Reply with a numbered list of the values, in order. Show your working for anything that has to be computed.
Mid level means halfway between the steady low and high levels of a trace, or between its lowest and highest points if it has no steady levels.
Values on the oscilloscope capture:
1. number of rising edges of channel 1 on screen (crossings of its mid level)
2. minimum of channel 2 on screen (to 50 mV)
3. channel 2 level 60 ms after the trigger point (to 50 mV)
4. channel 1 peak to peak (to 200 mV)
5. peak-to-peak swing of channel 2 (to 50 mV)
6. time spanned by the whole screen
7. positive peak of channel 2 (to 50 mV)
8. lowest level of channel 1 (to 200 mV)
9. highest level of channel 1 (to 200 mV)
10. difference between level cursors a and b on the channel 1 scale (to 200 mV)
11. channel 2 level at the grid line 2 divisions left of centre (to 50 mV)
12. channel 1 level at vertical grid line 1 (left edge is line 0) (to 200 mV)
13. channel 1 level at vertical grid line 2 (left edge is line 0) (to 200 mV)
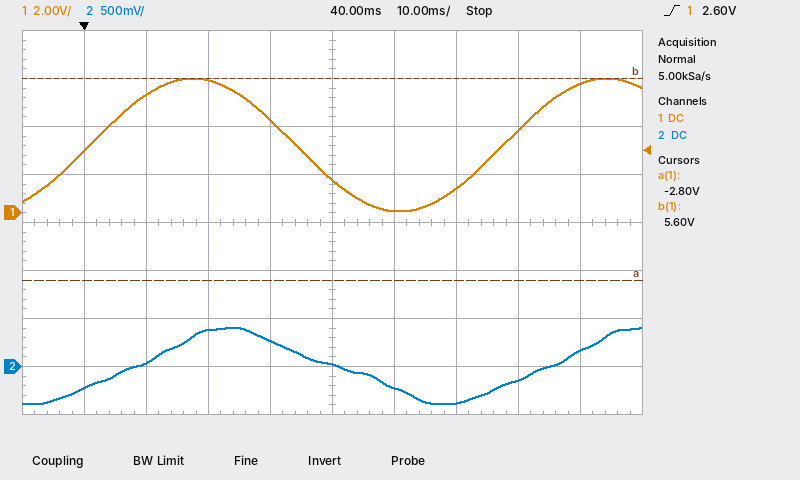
1. 2
2. -400 mV
3. -400 mV
4. 5.6 V − (0.0 V) = 5.6 V
5. 400 mV − (-400 mV) = 800 mV
6. 100 ms
7. 400 mV
8. 0.0 V
9. 5.6 V
10. 8.4 V
11. 400 mV
12. 2.6 V
13. 5.0 V
